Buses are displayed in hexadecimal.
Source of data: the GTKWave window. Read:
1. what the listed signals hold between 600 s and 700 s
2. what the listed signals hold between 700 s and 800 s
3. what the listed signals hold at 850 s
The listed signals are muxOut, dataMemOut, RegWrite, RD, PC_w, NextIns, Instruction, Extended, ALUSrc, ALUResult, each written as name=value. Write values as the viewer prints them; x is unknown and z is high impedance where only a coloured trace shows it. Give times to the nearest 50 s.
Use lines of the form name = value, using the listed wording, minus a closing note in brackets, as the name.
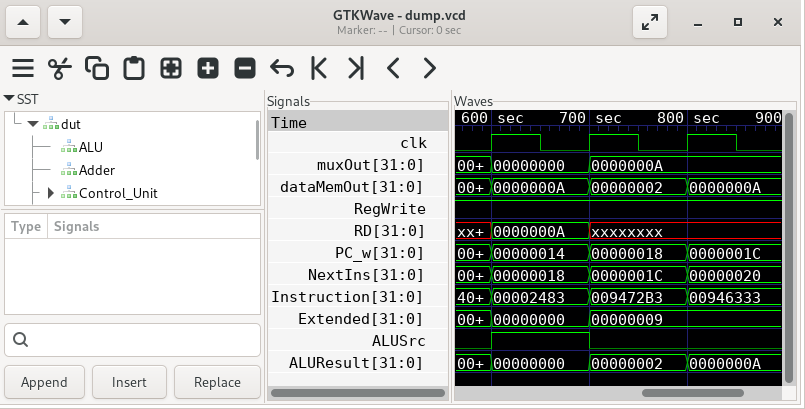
what the listed signals hold between 600 s and 700 s = muxOut=00000000, dataMemOut=0000000A, RegWrite=1, RD=0000000A, PC_w=00000014, NextIns=00000018, Instruction=00002483, Extended=00000000, ALUSrc=1, ALUResult=00000000
what the listed signals hold between 700 s and 800 s = muxOut=0000000A, dataMemOut=00000002, RegWrite=1, RD=xxxxxxxx, PC_w=00000018, NextIns=0000001C, Instruction=009472B3, Extended=00000009, ALUSrc=0, ALUResult=00000002
what the listed signals hold at 850 s = muxOut=0000000A, dataMemOut=0000000A, RegWrite=1, RD=xxxxxxxx, PC_w=0000001C, NextIns=00000020, Instruction=00946333, Extended=00000009, ALUSrc=0, ALUResult=0000000A
